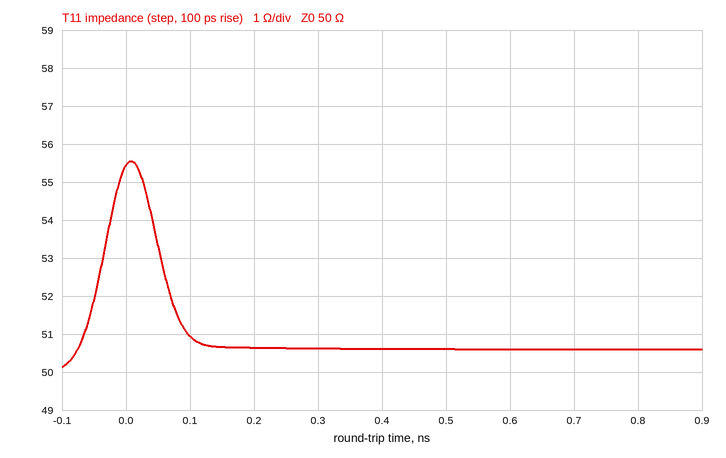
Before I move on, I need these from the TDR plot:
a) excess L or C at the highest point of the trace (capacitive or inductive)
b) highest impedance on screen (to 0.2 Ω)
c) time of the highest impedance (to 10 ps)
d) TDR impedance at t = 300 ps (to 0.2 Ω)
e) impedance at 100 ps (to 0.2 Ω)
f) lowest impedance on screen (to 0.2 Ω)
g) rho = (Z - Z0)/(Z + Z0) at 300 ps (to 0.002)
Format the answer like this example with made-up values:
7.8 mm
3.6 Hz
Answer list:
inductive
55.6 Ω
10 ps
50.6 Ω
51.0 Ω
50.2 Ω
+0.006
